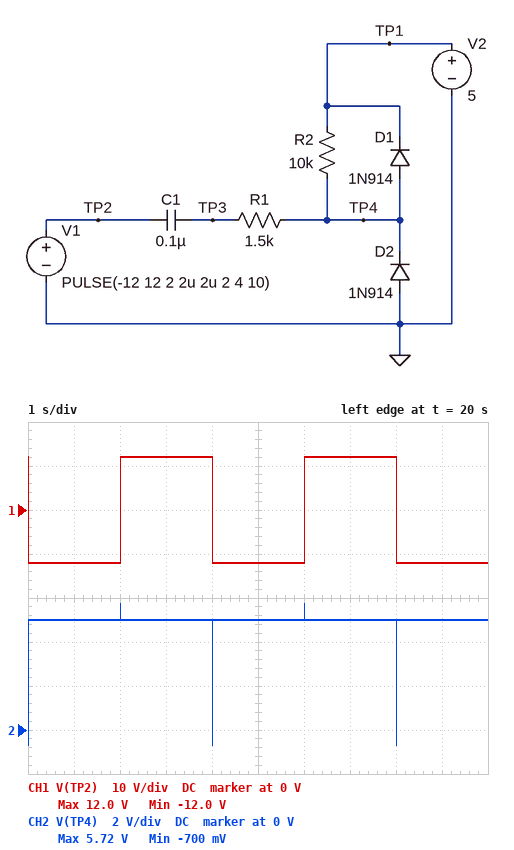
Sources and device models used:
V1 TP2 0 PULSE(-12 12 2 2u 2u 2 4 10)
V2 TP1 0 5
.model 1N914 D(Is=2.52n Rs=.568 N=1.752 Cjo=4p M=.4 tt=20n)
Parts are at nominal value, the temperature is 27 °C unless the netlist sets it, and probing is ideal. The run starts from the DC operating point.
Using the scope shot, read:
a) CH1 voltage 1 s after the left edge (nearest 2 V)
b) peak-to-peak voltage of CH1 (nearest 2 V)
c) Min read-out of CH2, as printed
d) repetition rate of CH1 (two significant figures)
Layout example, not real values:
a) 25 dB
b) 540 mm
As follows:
a) -12 V
b) 24 V
c) -700 mV
d) 250 mHz
